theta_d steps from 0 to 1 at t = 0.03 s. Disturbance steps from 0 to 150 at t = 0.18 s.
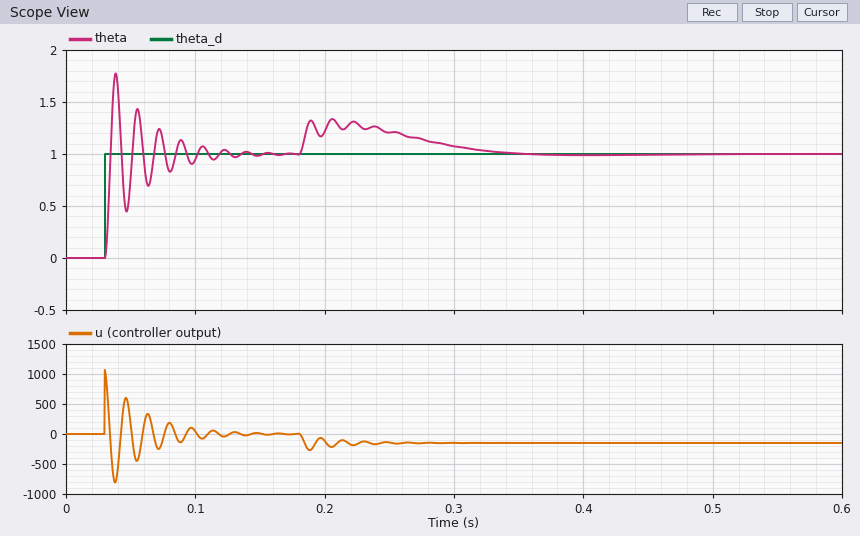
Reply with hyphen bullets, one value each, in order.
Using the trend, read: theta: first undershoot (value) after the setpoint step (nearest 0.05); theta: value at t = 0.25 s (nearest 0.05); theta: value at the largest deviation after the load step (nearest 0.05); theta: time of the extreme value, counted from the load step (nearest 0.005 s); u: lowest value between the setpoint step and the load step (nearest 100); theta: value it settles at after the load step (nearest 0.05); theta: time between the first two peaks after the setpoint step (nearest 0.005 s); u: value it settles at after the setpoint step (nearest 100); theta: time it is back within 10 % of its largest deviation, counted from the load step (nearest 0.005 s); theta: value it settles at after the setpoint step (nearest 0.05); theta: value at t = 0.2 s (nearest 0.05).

- 0.45
- 1.20
- 1.35
- 0.025 s
- -800
- 1.00
- 0.015 s
- 0
- 0.145 s
- 1.00
- 1.20
